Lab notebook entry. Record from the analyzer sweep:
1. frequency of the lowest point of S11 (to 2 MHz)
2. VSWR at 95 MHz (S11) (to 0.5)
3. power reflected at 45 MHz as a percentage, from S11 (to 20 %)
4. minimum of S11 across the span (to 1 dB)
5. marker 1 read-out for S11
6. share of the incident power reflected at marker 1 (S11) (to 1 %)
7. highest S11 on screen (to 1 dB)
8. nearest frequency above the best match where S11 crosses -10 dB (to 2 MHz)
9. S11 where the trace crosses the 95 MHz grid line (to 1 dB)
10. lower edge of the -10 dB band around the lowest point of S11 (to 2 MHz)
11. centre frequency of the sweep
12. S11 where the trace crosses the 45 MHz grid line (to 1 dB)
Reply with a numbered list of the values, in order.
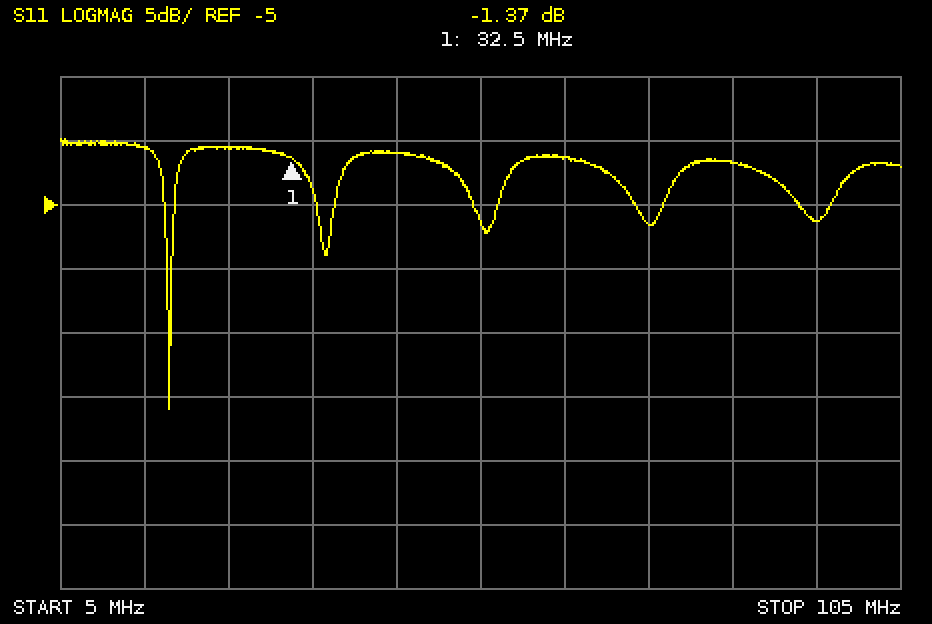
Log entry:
1. 18 MHz
2. 3.0
3. 80 %
4. -21 dB
5. -1.37 dB
6. 73 %
7. 0 dB
8. 18 MHz
9. -6 dB
10. 18 MHz
11. 55 MHz
12. -1 dB
